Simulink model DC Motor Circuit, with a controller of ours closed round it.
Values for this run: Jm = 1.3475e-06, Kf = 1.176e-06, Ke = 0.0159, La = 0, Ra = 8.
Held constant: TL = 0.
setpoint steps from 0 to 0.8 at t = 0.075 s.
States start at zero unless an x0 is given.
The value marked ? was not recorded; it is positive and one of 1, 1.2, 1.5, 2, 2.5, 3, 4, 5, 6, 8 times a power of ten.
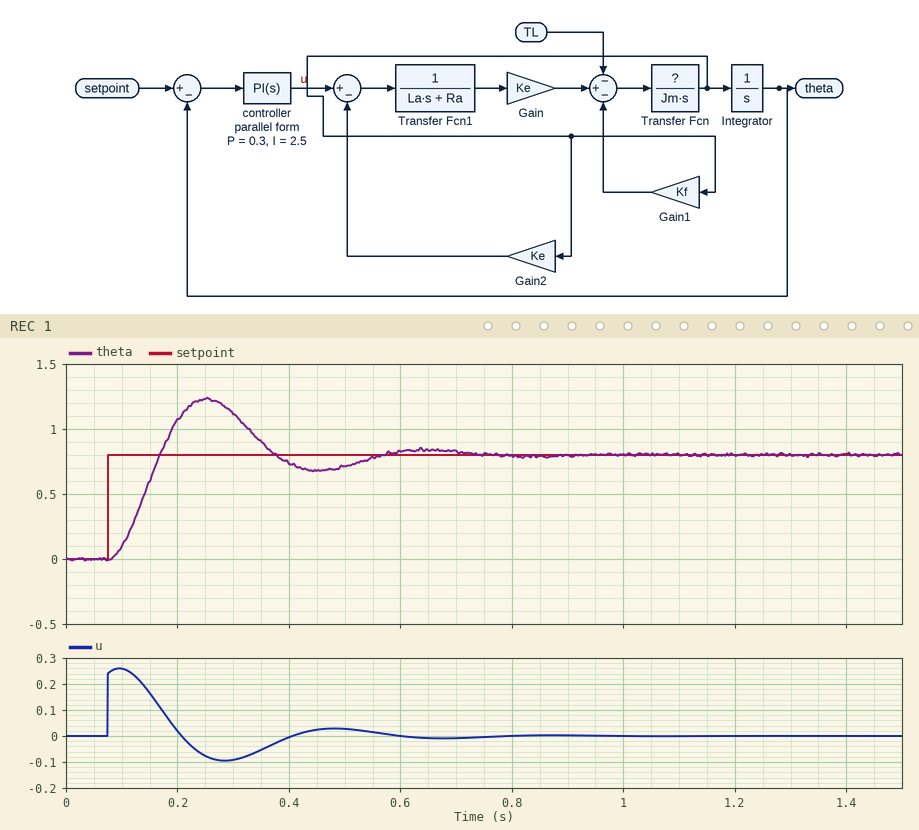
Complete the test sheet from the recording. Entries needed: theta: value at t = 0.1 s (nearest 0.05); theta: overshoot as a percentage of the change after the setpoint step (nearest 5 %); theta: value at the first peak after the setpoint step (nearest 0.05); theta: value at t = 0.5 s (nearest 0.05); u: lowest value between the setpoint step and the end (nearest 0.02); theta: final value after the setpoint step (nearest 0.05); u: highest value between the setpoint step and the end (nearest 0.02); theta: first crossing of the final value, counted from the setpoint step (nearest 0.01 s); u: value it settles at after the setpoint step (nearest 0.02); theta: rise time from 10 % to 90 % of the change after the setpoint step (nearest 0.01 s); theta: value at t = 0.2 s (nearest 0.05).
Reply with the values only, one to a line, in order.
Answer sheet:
0.10
55 %
1.25
0.70
-0.10
0.80
0.26
0.09 s
0.00
0.06 s
1.05
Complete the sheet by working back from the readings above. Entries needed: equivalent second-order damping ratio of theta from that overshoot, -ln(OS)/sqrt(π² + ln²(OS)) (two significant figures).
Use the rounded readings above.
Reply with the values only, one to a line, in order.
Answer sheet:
0.19
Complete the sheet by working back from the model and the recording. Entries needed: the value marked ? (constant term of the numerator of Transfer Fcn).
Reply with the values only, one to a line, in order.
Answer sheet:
1
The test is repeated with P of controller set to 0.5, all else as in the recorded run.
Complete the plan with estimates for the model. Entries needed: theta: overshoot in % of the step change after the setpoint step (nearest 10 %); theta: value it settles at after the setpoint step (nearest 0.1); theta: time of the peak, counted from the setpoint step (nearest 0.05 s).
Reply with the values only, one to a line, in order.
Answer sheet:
40 %
0.8
0.15 s
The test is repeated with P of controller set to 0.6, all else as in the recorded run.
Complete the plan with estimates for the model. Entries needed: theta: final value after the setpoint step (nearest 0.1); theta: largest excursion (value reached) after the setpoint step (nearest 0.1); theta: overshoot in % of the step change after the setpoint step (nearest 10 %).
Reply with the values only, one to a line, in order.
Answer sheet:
0.8
1.1
40 %
